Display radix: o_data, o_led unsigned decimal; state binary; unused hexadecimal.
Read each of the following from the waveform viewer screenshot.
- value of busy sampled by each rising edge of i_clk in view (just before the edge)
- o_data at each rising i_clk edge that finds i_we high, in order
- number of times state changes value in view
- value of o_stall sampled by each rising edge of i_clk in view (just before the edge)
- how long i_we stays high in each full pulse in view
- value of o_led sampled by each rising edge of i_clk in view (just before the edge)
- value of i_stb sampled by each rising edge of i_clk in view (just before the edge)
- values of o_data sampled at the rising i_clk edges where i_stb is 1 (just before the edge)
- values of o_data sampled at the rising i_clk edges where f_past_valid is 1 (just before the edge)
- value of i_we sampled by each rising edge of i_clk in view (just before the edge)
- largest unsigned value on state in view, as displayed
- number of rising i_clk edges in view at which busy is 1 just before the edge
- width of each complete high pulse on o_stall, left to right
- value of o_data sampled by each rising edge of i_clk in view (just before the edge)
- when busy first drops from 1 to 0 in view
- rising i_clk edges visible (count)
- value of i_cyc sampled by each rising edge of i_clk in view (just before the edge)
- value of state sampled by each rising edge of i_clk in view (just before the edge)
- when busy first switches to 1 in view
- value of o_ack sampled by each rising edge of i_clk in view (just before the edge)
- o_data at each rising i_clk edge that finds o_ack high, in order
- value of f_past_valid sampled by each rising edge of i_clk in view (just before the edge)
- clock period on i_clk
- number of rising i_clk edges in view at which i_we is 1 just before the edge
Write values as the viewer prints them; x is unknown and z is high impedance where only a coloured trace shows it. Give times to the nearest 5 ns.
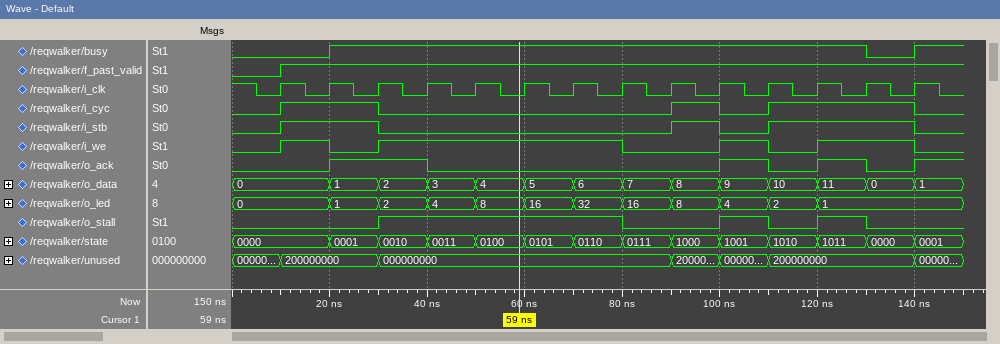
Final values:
0 0 1 1 1 1 1 1 1 1 1 1 1 0
0, 2, 3, 4, 5, 6, 9, 11, 0
13
0 0 0 1 1 1 1 1 0 0 1 0 1 0
10 ns, 50 ns, 10 ns, 20 ns
0, 0, 1, 2, 4, 8, 16, 32, 16, 8, 4, 2, 1, 1
0 1 1 0 0 0 0 0 0 1 0 1 1 1
0, 1, 8, 10, 11, 0
0, 1, 2, 3, 4, 5, 6, 7, 8, 9, 10, 11, 0
0 1 0 1 1 1 1 1 0 0 1 0 1 1
1011
11
50 ns, 10 ns, 10 ns
0, 0, 1, 2, 3, 4, 5, 6, 7, 8, 9, 10, 11, 0
130 ns
14
0 1 1 0 0 0 0 0 0 1 0 1 1 1
0000, 0000, 0001, 0010, 0011, 0100, 0101, 0110, 0111, 1000, 1001, 1010, 1011, 0000
20 ns
0 0 1 1 0 0 0 0 0 0 1 0 1 0
1, 2, 9, 11
0 1 1 1 1 1 1 1 1 1 1 1 1 1
10 ns
9
